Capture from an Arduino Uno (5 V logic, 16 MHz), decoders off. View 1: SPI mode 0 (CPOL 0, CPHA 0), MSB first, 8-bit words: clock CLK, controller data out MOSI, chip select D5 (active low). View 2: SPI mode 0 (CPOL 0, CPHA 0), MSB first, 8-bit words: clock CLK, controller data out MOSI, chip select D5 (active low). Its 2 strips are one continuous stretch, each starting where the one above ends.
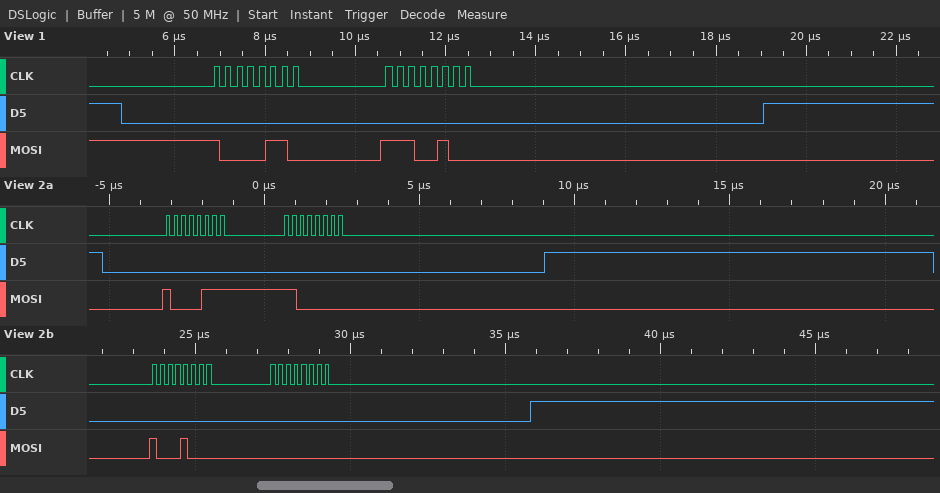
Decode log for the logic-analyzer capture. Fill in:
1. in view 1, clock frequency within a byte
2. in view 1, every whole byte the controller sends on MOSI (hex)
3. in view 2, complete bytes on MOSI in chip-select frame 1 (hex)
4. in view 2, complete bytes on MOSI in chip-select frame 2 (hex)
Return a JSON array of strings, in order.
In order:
["4 MHz", "86 E4", "0x87 0xC0", "0x88 0x00"]
